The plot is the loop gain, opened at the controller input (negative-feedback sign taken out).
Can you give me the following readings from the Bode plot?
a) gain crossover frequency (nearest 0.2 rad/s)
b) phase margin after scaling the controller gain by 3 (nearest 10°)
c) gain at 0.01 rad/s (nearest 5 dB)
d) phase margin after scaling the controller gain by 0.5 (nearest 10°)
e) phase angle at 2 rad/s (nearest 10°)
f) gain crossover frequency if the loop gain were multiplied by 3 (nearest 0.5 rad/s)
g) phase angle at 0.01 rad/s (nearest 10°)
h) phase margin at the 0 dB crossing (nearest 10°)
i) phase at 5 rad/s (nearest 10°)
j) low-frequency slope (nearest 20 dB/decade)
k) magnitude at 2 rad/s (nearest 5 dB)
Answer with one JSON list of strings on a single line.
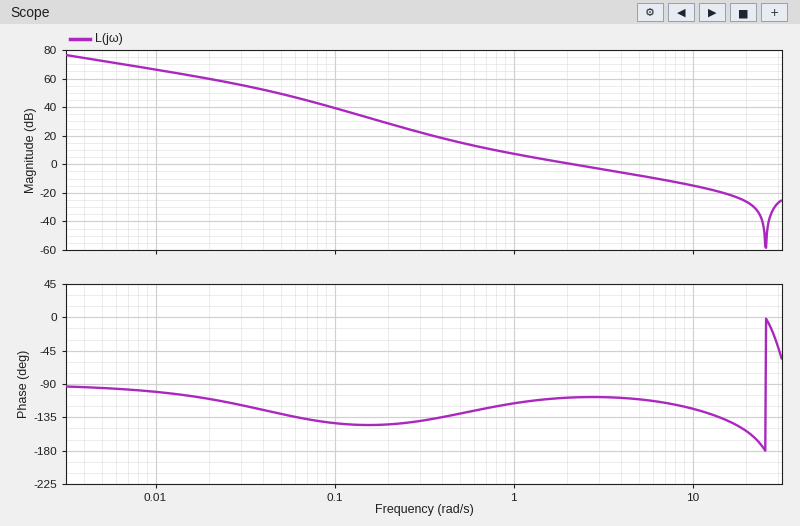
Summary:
["2.2 rad/s", "70°", "65 dB", "70°", "-110°", "6.0 rad/s", "-100°", "70°", "-110°", "-20 dB/decade", "0 dB"]
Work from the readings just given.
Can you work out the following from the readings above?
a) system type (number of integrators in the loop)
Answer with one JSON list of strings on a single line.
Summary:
["1"]
